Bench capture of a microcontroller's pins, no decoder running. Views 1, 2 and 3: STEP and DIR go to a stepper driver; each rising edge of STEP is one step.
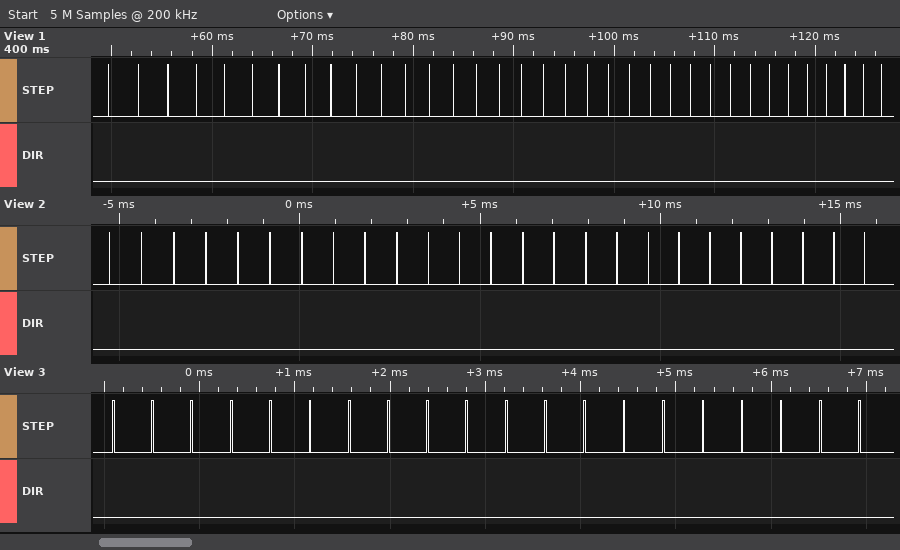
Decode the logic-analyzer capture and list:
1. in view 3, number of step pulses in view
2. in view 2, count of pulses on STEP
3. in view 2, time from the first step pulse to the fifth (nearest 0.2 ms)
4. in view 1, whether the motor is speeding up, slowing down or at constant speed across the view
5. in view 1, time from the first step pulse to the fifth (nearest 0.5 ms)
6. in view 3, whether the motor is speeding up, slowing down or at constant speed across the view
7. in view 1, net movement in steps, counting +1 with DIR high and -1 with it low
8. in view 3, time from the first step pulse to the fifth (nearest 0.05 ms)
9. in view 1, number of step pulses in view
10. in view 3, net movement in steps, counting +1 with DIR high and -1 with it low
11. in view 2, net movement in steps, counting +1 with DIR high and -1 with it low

20
25
3.6 ms
speeding up
11.5 ms
constant speed
-35
1.65 ms
35
-20
-25
